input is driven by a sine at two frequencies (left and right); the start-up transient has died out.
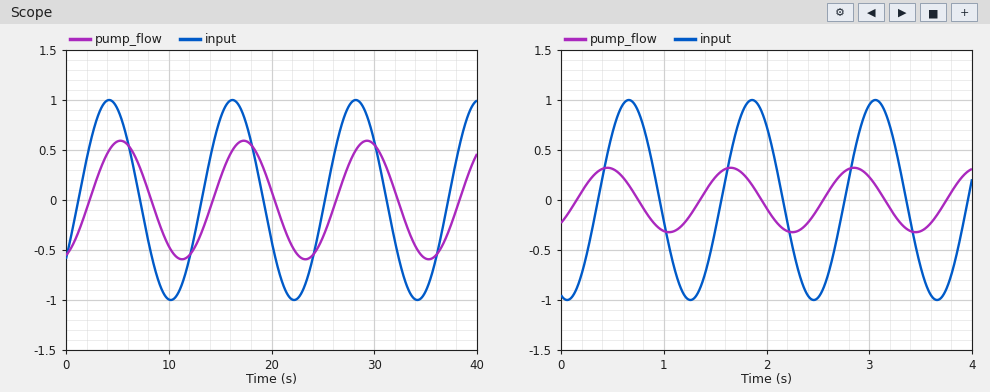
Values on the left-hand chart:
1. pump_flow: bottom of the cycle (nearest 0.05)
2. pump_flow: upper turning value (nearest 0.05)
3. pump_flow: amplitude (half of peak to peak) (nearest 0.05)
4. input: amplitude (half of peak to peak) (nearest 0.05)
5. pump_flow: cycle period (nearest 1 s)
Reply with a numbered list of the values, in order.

1. -0.60
2. 0.60
3. 0.60
4. 1.00
5. 12 s
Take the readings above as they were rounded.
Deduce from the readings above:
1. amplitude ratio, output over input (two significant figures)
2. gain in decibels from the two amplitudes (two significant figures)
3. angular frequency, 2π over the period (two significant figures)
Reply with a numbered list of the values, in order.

1. 0.60
2. -4.4 dB
3. 0.52 rad/s
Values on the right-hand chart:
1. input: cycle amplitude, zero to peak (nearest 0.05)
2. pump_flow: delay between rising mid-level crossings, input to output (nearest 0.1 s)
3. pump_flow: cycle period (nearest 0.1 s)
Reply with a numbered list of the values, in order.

1. 1.00
2. 1.0 s
3. 1.2 s
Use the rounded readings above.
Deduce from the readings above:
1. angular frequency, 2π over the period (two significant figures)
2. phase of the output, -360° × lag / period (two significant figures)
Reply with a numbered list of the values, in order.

1. 5.2 rad/s
2. -300°
